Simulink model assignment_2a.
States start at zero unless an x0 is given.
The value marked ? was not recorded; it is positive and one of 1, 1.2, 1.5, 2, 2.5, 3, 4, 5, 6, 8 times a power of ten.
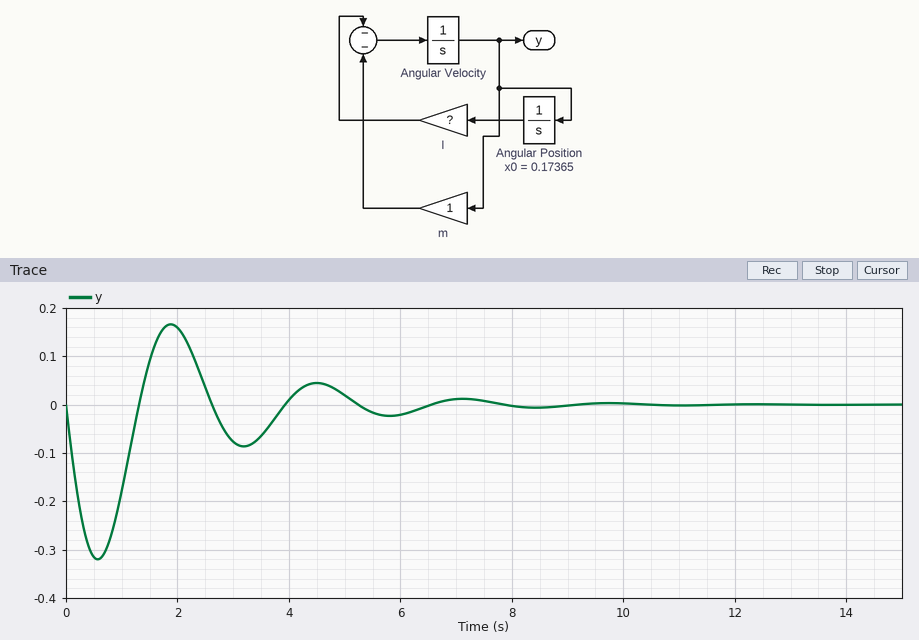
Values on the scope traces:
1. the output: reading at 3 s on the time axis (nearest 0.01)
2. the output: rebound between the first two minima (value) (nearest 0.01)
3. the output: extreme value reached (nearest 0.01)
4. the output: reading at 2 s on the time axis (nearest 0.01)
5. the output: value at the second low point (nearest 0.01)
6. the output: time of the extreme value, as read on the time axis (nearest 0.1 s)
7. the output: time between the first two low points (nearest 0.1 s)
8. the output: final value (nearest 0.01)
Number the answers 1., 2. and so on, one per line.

1. -0.08
2. 0.17
3. -0.32
4. 0.16
5. -0.09
6. 0.6 s
7. 2.6 s
8. 0.00
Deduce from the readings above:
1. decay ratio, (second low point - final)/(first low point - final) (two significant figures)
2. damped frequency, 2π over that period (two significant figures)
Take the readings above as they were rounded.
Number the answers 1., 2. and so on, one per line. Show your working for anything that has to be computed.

1. (-0.09 - 0) / (-0.32 - 0) = 0.28
2. 2π / 2.6 = 2.4 rad/s
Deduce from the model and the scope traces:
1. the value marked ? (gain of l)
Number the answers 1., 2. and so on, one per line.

1. 6
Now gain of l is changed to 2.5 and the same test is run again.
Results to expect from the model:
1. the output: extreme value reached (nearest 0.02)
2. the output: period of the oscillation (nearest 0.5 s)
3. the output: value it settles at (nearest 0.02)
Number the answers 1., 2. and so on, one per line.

1. -0.18
2. 4.0 s
3. 0.00
